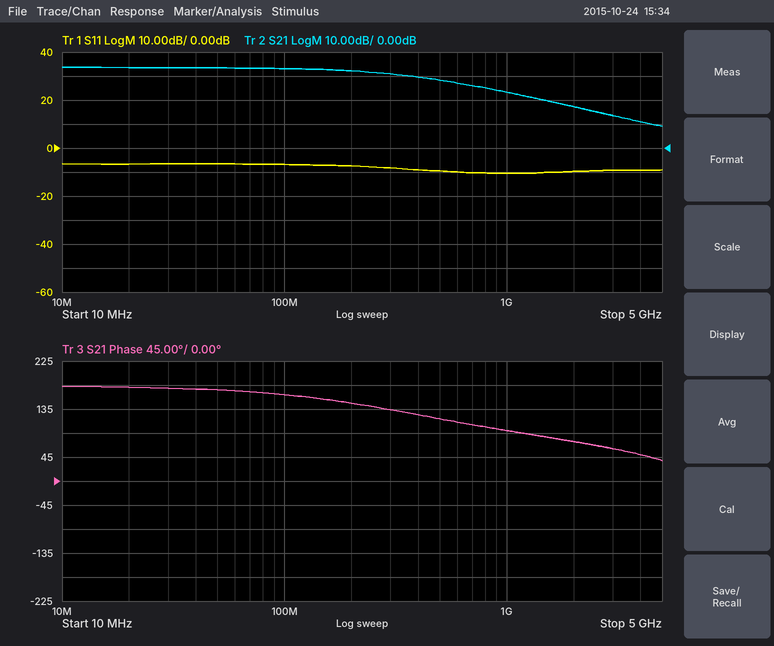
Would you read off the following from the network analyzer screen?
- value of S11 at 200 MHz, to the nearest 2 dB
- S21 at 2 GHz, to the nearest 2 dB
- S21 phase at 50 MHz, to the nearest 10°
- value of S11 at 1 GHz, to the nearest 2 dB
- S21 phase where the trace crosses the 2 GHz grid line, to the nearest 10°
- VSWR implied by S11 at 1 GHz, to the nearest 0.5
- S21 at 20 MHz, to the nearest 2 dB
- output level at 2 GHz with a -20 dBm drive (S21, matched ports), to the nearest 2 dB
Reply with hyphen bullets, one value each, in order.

- -8 dB
- 18 dB
- 170°
- -10 dB
- 70°
- 2.0
- 34 dB
- -2 dBm
